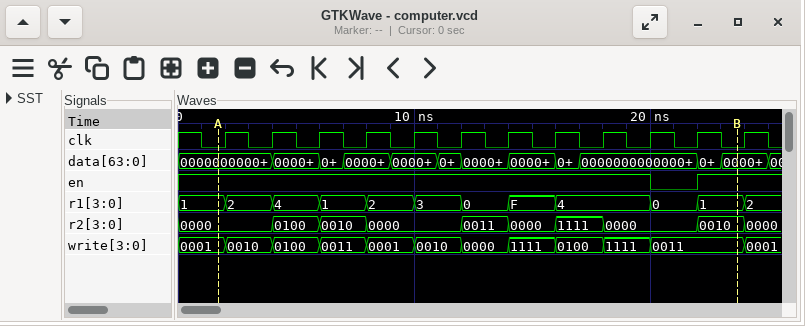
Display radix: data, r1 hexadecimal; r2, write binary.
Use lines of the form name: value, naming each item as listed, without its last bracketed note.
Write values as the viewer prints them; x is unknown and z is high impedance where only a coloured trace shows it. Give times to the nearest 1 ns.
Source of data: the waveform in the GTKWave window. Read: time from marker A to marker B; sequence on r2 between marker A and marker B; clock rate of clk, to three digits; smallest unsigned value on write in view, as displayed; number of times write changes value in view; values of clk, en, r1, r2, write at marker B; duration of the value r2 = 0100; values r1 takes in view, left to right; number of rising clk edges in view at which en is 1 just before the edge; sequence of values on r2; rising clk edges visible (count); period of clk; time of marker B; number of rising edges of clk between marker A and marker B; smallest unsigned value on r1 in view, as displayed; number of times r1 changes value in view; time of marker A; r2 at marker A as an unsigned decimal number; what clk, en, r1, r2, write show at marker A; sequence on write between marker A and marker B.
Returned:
time from marker A to marker B: 22 ns
sequence on r2 between marker A and marker B: 0000, 0100, 0010, 0000, 0011, 0000, 1111, 0000, 0010
clock rate of clk, to three digits: 500 MHz
smallest unsigned value on write in view, as displayed: 0000
number of times write changes value in view: 11
values of clk, en, r1, r2, write at marker B: clk=0, en=1, r1=1, r2=0010, write=0011
duration of the value r2 = 0100: 2 ns
values r1 takes in view, left to right: 1, 2, 4, 1, 2, 3, 0, F, 4, 0, 1, 2
number of rising clk edges in view at which en is 1 just before the edge: 11
sequence of values on r2: 0000, 0100, 0010, 0000, 0011, 0000, 1111, 0000, 0010, 0000
rising clk edges visible: 12
period of clk: 2 ns
time of marker B: 24 ns
number of rising edges of clk between marker A and marker B: 11
smallest unsigned value on r1 in view, as displayed: 0
number of times r1 changes value in view: 11
time of marker A: 2 ns
r2 at marker A as an unsigned decimal number: 0
what clk, en, r1, r2, write show at marker A: clk=0, en=1, r1=1, r2=0000, write=0001
sequence on write between marker A and marker B: 0001, 0010, 0100, 0011, 0001, 0010, 0000, 1111, 0100, 1111, 0011
